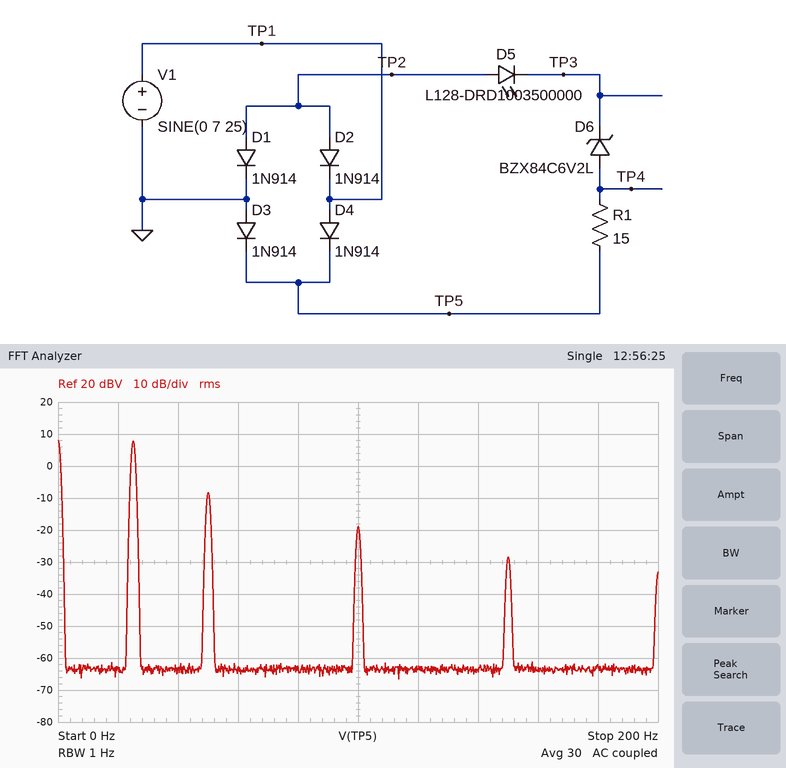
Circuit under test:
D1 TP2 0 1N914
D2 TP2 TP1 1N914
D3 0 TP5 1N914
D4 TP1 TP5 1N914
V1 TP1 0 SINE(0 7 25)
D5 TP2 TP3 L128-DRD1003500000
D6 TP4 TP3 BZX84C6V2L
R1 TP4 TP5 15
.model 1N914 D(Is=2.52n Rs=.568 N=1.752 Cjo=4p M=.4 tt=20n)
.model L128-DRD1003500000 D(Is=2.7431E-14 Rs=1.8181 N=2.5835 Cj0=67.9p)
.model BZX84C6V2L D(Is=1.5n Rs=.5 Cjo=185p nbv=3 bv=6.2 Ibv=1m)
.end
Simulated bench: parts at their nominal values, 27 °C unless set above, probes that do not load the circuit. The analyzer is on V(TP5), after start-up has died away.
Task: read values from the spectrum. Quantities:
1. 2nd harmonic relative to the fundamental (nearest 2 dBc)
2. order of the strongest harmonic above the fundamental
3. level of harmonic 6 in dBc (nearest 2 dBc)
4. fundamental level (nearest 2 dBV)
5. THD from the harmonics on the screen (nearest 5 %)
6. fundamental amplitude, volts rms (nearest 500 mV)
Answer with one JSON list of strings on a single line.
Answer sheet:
["-16 dBc", "2", "-36 dBc", "8 dBV", "15 %", "2.5 V"]
